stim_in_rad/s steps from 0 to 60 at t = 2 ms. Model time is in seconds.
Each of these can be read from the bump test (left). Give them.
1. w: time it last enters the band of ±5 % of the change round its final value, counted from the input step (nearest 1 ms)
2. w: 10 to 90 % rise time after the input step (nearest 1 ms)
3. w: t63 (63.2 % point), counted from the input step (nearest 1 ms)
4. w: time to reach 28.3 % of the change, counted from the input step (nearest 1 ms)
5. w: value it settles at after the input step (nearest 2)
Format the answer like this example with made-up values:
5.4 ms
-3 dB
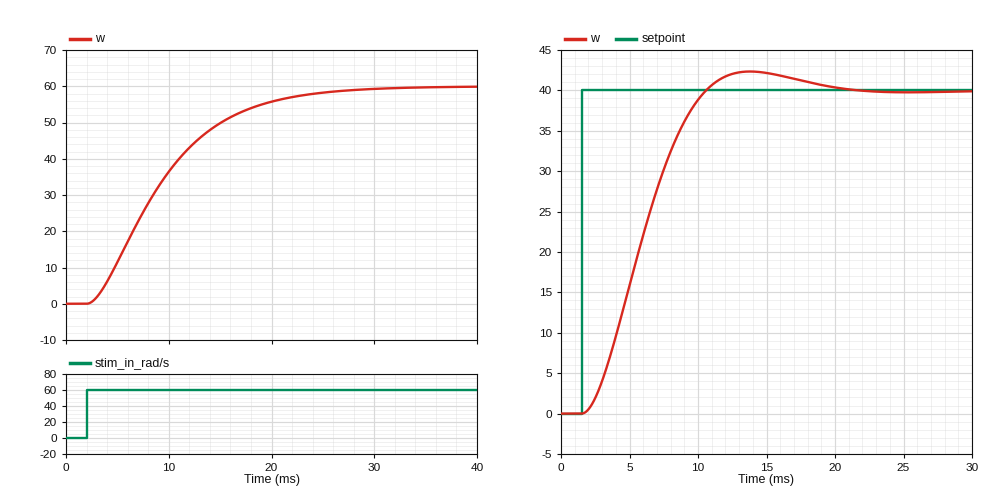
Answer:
20 ms
14 ms
8 ms
4 ms
60
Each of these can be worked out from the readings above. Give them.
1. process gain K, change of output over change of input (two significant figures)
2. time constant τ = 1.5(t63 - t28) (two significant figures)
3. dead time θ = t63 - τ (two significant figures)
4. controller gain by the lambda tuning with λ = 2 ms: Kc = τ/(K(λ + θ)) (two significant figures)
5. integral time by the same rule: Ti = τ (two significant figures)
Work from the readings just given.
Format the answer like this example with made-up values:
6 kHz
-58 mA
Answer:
1.0
6.0 ms
2.0 ms
1.5
6.0 ms
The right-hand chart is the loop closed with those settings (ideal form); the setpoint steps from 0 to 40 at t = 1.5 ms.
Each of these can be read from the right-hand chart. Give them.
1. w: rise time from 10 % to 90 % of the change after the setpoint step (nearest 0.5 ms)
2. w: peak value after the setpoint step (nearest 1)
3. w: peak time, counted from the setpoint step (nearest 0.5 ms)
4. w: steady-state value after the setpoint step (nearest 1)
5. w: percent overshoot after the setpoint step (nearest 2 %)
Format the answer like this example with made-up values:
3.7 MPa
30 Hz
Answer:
6.0 ms
42
12.5 ms
40
6 %
